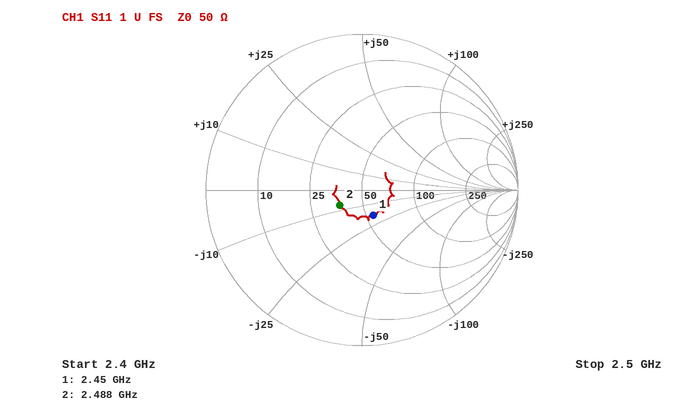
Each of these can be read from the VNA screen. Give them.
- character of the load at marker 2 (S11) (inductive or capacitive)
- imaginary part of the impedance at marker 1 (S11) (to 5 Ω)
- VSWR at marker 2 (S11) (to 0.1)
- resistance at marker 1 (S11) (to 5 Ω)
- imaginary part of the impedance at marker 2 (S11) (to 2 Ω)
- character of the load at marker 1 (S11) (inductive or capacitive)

capacitive
-20 Ω
1.4
55 Ω
-8 Ω
capacitive
